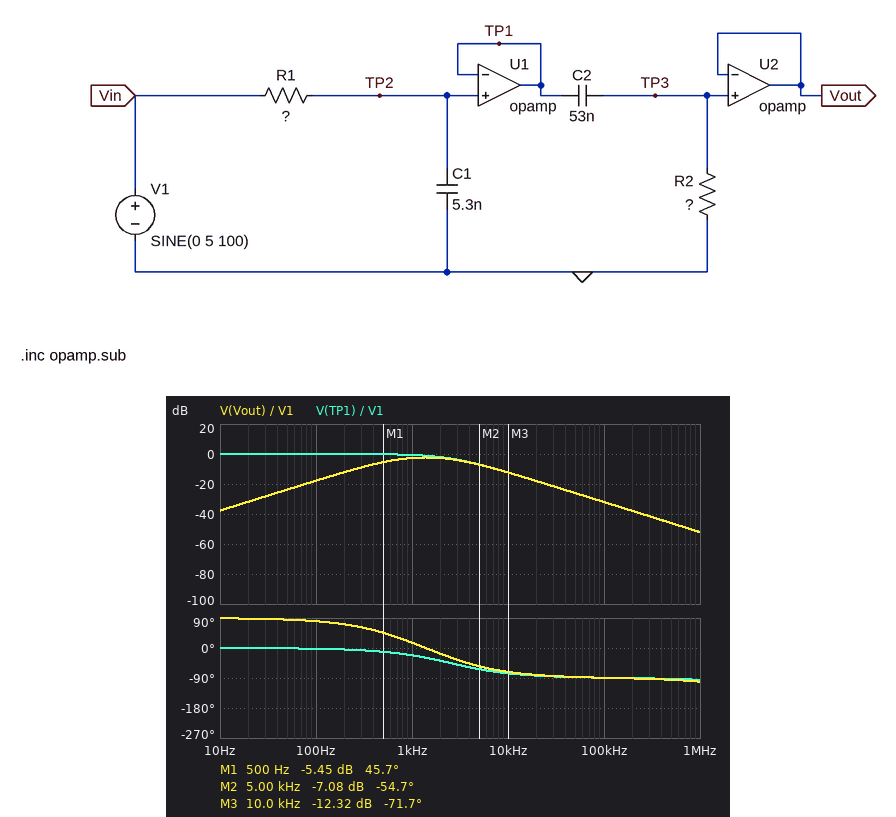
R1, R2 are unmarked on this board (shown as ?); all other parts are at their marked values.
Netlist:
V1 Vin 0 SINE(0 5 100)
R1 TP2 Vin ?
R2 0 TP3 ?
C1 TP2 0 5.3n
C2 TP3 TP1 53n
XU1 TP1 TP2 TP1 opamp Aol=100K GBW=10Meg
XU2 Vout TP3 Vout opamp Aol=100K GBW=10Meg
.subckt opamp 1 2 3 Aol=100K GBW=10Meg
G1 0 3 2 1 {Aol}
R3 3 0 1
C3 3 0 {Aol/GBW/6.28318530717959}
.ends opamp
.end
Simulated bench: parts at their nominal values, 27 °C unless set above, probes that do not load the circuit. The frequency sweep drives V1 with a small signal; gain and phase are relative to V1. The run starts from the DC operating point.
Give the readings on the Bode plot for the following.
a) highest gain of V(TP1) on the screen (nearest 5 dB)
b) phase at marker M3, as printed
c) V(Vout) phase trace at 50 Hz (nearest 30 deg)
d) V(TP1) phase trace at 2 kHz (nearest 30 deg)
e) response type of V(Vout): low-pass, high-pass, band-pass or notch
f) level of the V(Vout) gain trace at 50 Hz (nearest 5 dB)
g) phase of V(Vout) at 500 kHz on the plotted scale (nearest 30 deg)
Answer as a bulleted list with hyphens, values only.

- 0 dB
- -71.7 deg
- 90 deg
- -30 deg
- band-pass
- -25 dB
- -90 deg
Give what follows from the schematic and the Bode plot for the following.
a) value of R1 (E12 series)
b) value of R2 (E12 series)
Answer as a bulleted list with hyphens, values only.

- 12 kΩ
- 3.9 kΩ
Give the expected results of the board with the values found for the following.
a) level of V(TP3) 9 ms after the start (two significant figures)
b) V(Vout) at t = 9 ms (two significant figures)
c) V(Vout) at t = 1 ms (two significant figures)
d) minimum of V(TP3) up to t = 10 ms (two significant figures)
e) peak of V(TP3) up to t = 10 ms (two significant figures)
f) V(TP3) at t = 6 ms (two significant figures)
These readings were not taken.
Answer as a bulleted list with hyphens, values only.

- 450 mV
- 450 mV
- 570 mV
- -640 mV
- 630 mV
- -580 mV
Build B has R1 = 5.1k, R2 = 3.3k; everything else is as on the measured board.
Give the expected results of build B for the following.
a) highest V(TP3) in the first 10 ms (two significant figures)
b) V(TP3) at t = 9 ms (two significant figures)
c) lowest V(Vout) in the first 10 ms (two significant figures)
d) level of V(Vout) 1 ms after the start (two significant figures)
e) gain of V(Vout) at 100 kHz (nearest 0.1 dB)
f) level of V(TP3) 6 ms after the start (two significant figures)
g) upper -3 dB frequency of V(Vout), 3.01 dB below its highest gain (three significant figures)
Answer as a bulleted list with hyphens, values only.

- 540 mV
- 400 mV
- -550 mV
- 480 mV
- -24.6 dB
- -480 mV
- 7.51 kHz
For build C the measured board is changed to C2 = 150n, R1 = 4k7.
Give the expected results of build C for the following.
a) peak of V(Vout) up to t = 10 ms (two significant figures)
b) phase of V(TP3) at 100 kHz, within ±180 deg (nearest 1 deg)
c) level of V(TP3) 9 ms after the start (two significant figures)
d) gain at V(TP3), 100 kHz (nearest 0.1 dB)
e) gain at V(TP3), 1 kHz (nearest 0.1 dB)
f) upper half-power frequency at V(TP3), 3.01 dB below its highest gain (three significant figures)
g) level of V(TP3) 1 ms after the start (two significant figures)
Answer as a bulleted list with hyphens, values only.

- 1.6 V
- -87 deg
- 940 mV
- -23.9 dB
- -0.4 dB
- 6.91 kHz
- 1.4 V
